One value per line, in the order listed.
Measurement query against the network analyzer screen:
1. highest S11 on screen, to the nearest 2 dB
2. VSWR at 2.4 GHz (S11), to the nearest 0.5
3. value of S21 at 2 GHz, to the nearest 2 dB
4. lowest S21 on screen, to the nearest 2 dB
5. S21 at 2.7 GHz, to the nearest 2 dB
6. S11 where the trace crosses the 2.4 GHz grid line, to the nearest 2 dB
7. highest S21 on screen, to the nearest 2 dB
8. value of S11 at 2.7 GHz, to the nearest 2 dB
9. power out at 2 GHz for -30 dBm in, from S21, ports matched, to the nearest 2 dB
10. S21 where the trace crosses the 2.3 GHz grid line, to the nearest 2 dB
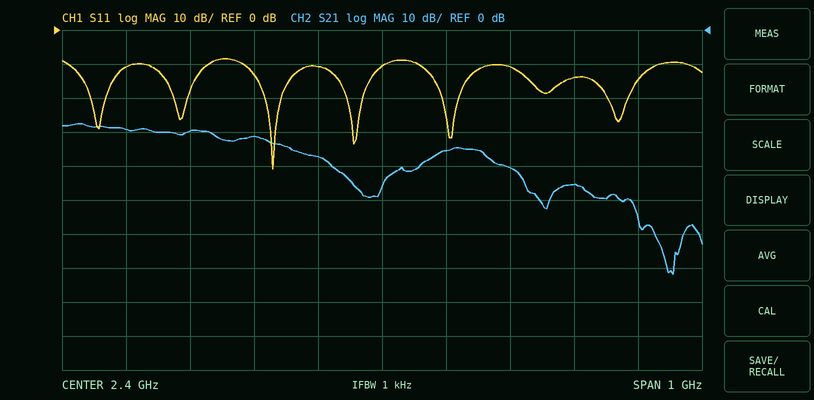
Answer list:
-8 dB
2.0
-30 dB
-72 dB
-46 dB
-10 dB
-28 dB
-14 dB
-60 dBm
-38 dB
